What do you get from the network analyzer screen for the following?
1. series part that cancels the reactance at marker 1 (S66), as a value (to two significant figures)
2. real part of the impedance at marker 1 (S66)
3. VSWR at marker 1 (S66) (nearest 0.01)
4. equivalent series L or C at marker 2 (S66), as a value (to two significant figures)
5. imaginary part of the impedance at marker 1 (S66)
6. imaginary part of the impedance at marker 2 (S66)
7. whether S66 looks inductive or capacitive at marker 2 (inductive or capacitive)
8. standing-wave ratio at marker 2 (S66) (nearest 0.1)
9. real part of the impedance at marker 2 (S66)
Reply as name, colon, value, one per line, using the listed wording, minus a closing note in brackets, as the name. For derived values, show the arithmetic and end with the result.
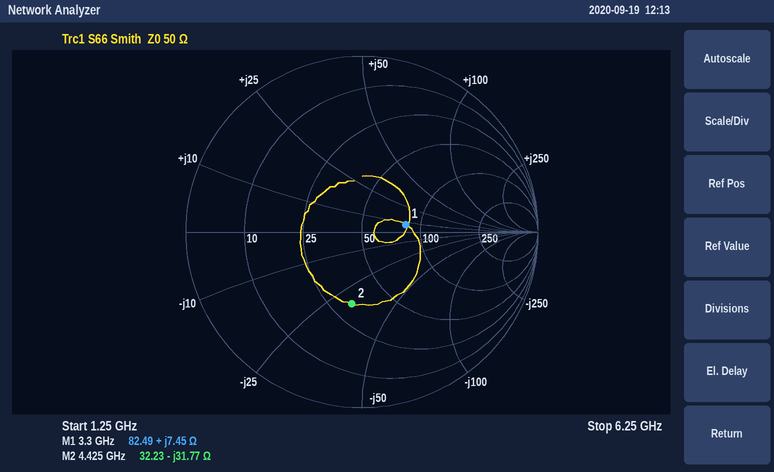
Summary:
series part that cancels the reactance at marker 1 (S66), as a value: C = 1/(2π × 3.3 GHz × 7.45 Ω) ≈ 6.5 pF
real part of the impedance at marker 1: 82.49 Ω
VSWR at marker 1 (S66): 1.67
equivalent series L or C at marker 2 (S66), as a value: C = 1/(2π × 4.425 GHz × 31.77 Ω) ≈ 1.1 pF
imaginary part of the impedance at marker 1: +7.45 Ω
imaginary part of the impedance at marker 2: -31.77 Ω
whether S66 looks inductive or capacitive at marker 2: capacitive
standing-wave ratio at marker 2 (S66): 2.4
real part of the impedance at marker 2: 32.23 Ω
